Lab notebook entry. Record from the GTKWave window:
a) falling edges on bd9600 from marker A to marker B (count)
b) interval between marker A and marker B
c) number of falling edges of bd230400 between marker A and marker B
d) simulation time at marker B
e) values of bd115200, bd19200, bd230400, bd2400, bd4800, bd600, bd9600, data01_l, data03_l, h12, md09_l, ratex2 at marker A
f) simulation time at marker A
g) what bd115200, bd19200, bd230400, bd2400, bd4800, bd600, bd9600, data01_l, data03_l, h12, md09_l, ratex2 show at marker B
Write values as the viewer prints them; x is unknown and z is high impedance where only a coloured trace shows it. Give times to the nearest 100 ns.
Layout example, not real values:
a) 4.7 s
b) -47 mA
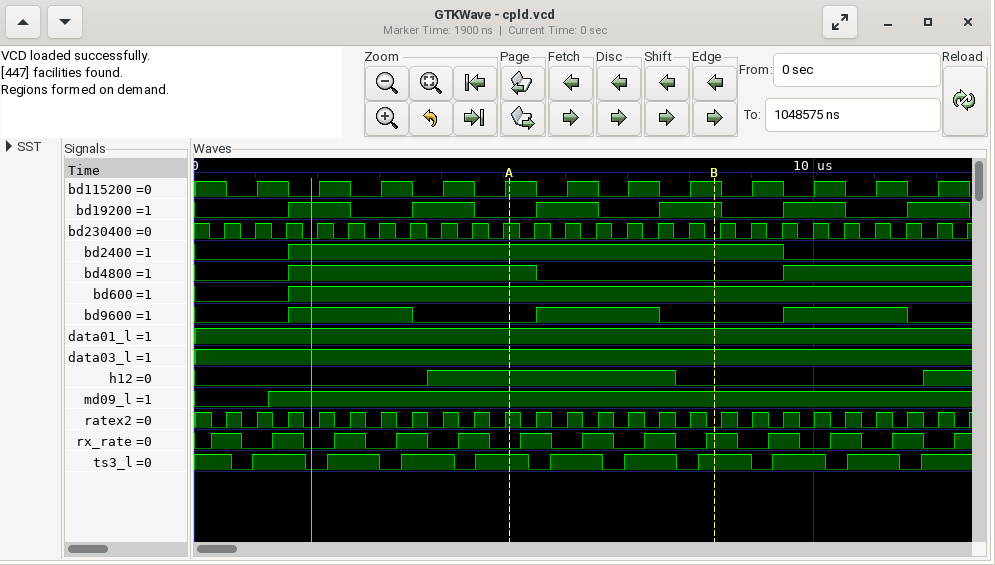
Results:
a) 1
b) 3300 ns
c) 7
d) 8400 ns
e) bd115200=1, bd19200=0, bd230400=1, bd2400=1, bd4800=1, bd600=1, bd9600=0, data01_l=1, data03_l=1, h12=1, md09_l=1, ratex2=1
f) 5100 ns
g) bd115200=1, bd19200=1, bd230400=0, bd2400=1, bd4800=0, bd600=1, bd9600=0, data01_l=1, data03_l=1, h12=0, md09_l=1, ratex2=0
